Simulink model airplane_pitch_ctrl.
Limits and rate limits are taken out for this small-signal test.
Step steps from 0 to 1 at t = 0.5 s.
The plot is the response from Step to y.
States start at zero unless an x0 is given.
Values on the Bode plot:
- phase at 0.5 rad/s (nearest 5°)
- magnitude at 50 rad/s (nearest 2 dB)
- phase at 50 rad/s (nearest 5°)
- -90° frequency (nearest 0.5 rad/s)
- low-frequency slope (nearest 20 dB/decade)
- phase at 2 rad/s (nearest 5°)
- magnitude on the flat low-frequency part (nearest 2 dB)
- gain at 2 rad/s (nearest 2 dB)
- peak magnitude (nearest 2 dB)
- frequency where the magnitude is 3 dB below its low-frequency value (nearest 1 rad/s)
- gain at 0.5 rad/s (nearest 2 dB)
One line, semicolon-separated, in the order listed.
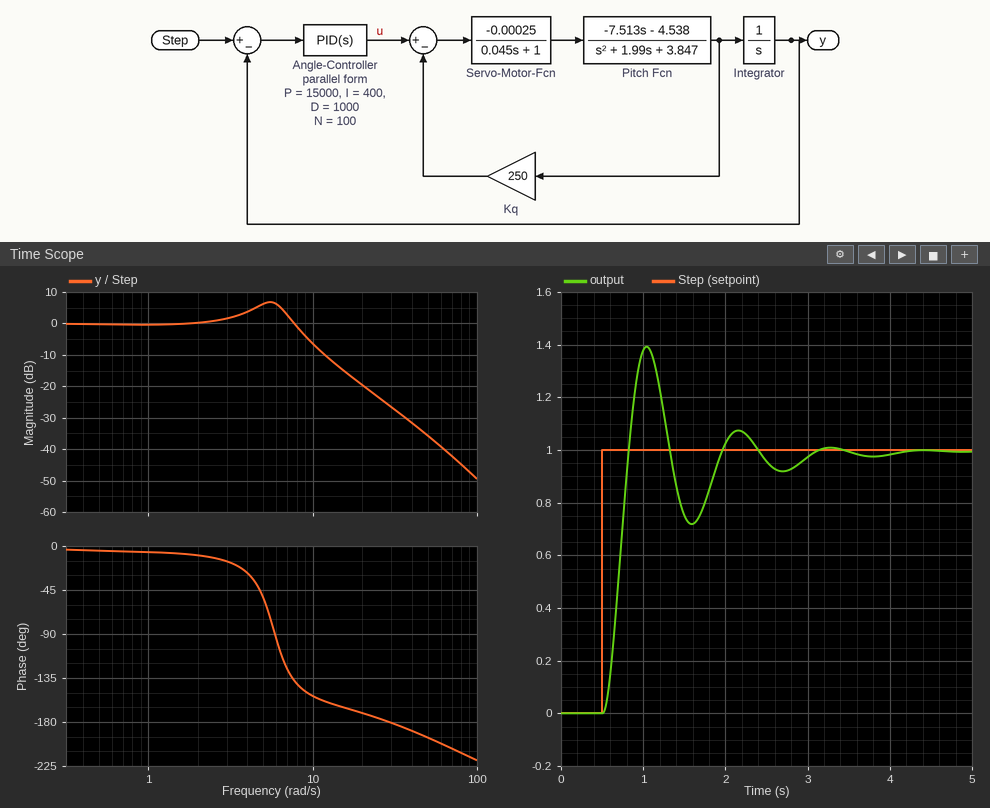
-5°; -36 dB; -195°; 6.0 rad/s; 0 dB/decade; -10°; 0 dB; 0 dB; 6 dB; 9 rad/s; 0 dB
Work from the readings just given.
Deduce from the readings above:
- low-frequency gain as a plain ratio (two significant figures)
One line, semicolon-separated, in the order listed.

1.0
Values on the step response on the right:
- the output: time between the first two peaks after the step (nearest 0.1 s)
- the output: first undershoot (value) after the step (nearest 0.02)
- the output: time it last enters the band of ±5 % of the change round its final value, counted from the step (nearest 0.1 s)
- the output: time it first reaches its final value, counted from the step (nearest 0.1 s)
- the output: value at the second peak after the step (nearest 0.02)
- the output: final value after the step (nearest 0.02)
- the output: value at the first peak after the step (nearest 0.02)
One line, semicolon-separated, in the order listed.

1.1 s; 0.72; 2.4 s; 0.3 s; 1.08; 1.00; 1.40
